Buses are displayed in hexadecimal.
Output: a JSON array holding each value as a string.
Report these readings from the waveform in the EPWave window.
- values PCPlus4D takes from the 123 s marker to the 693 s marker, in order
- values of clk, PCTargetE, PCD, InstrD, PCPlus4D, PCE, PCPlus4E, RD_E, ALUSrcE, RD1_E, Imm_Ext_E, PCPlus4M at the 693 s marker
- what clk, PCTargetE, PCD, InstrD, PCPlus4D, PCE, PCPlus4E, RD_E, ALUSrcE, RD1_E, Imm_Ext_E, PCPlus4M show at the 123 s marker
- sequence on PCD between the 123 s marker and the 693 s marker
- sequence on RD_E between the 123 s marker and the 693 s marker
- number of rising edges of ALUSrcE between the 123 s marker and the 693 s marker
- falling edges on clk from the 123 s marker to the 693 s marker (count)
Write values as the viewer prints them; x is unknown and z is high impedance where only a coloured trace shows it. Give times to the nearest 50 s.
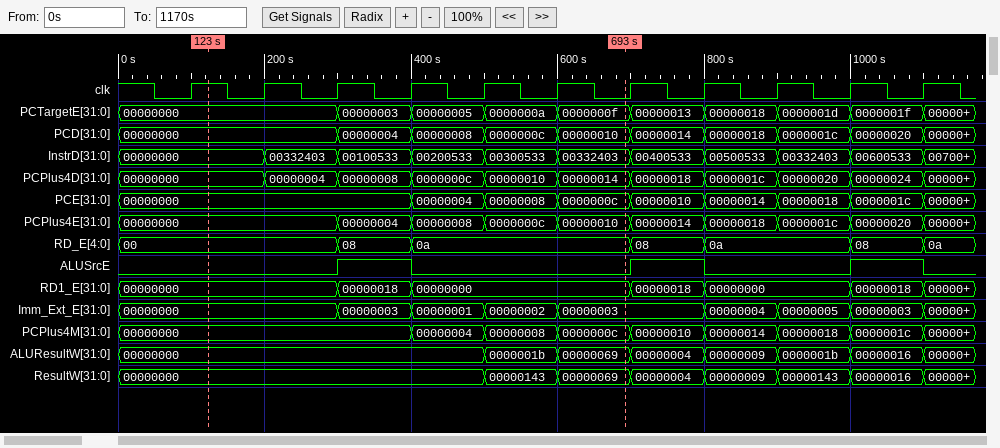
["00000000, 00000004, 00000008, 0000000c, 00000010, 00000014", "clk=0, PCTargetE=0000000f, PCD=00000010, InstrD=00332403, PCPlus4D=00000014, PCE=0000000c, PCPlus4E=00000010, RD_E=0a, ALUSrcE=0, RD1_E=00000000, Imm_Ext_E=00000003, PCPlus4M=0000000c", "clk=1, PCTargetE=00000000, PCD=00000000, InstrD=00000000, PCPlus4D=00000000, PCE=00000000, PCPlus4E=00000000, RD_E=00, ALUSrcE=0, RD1_E=00000000, Imm_Ext_E=00000000, PCPlus4M=00000000", "00000000, 00000004, 00000008, 0000000c, 00000010", "00, 08, 0a", "1", "6"]
